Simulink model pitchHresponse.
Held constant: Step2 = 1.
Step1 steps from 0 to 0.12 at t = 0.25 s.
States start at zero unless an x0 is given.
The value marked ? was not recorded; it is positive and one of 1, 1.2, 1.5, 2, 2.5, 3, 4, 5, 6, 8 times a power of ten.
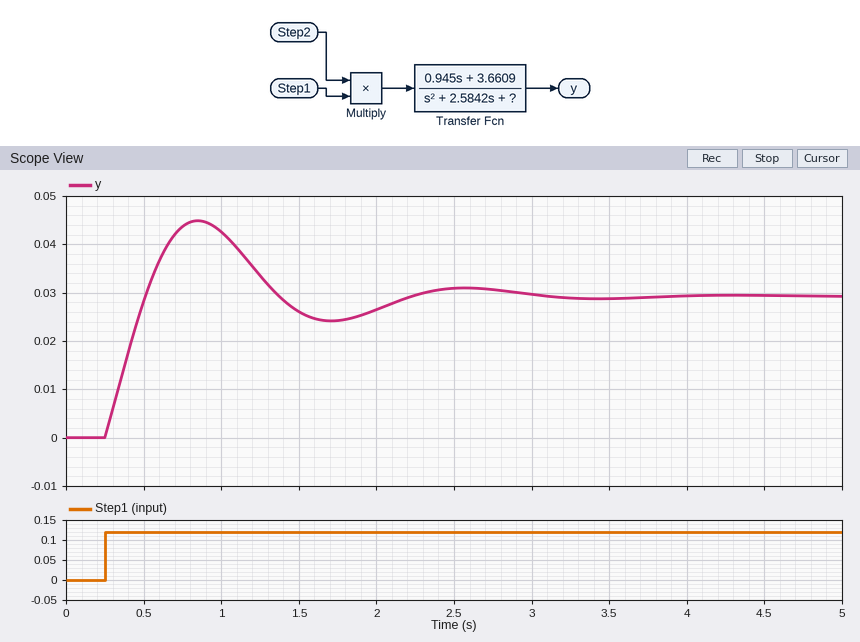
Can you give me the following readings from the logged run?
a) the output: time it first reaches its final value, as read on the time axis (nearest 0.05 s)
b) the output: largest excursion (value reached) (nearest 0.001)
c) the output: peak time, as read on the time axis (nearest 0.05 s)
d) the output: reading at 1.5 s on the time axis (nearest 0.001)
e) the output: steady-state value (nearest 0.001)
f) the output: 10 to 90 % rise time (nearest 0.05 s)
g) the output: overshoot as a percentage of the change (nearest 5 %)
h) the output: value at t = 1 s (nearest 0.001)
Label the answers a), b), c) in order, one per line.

a) 0.50 s
b) 0.045
c) 0.85 s
d) 0.026
e) 0.029
f) 0.20 s
g) 55 %
h) 0.043
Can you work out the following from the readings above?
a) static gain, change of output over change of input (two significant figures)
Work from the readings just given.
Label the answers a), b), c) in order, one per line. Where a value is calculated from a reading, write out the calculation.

a) (0.029 - 0) / (0.12 - 0) = 0.24
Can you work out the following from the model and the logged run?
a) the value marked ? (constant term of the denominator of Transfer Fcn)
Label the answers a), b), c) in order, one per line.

a) 15
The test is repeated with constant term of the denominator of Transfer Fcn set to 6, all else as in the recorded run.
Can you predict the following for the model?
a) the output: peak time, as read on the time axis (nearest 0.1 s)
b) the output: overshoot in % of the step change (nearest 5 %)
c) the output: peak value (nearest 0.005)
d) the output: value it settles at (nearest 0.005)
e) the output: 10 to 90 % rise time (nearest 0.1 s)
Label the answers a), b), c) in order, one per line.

a) 1.4 s
b) 20 %
c) 0.085
d) 0.075
e) 0.5 s
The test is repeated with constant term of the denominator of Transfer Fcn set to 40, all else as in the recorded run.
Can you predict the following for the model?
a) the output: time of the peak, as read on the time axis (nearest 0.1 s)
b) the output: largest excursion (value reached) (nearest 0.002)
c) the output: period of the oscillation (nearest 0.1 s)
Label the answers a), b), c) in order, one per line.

a) 0.6 s
b) 0.024
c) 1.0 s
